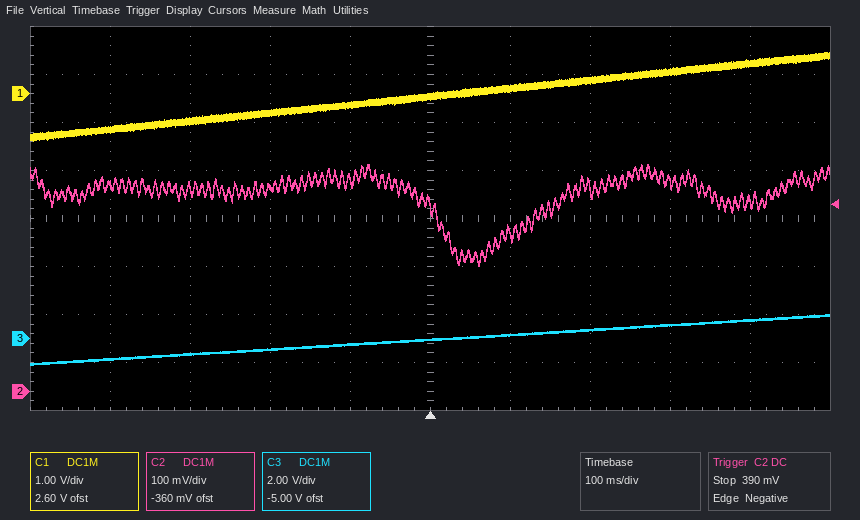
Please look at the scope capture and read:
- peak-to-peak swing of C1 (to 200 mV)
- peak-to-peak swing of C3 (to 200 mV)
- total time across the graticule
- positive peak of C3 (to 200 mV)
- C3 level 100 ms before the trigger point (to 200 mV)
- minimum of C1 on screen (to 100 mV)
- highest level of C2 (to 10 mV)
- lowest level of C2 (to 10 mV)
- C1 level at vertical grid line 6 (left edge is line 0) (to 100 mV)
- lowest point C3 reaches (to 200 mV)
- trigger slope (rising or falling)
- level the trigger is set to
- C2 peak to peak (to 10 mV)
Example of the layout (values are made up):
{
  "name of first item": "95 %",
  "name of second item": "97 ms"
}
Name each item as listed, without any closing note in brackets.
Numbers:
{
  "peak-to-peak swing of C1": "1.8 V",
  "peak-to-peak swing of C3": "2.0 V",
  "total time across the graticule": "1 s",
  "positive peak of C3": "1.0 V",
  "C3 level 100 ms before the trigger point": "-200 mV",
  "minimum of C1 on screen": "-1.0 V",
  "highest level of C2": "470 mV",
  "lowest level of C2": "260 mV",
  "C1 level at vertical grid line 6 (left edge is line 0)": "100 mV",
  "lowest point C3 reaches": "-1.0 V",
  "trigger slope": "falling",
  "level the trigger is set to": "390 mV",
  "C2 peak to peak": "210 mV"
}
